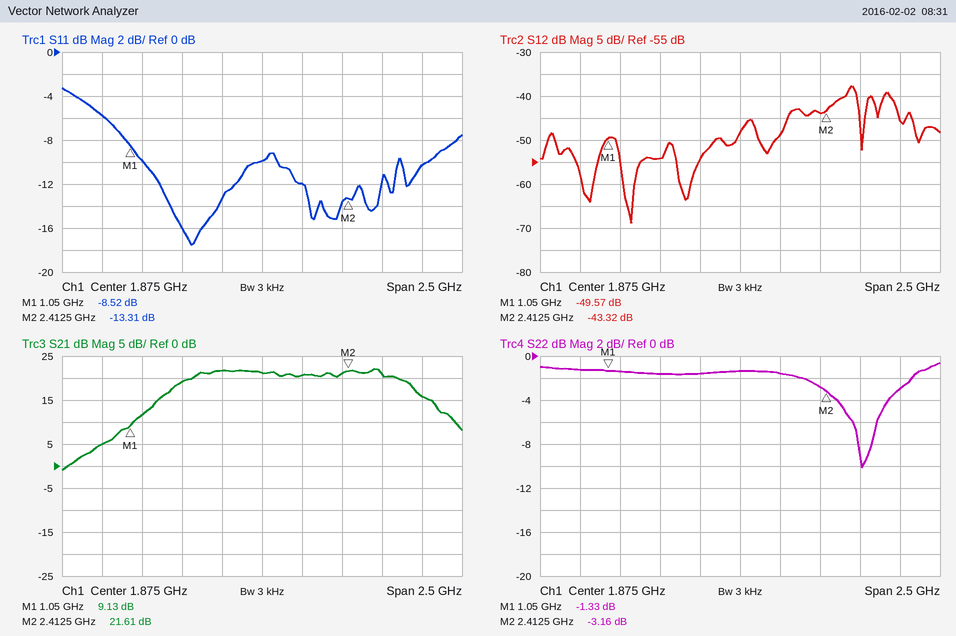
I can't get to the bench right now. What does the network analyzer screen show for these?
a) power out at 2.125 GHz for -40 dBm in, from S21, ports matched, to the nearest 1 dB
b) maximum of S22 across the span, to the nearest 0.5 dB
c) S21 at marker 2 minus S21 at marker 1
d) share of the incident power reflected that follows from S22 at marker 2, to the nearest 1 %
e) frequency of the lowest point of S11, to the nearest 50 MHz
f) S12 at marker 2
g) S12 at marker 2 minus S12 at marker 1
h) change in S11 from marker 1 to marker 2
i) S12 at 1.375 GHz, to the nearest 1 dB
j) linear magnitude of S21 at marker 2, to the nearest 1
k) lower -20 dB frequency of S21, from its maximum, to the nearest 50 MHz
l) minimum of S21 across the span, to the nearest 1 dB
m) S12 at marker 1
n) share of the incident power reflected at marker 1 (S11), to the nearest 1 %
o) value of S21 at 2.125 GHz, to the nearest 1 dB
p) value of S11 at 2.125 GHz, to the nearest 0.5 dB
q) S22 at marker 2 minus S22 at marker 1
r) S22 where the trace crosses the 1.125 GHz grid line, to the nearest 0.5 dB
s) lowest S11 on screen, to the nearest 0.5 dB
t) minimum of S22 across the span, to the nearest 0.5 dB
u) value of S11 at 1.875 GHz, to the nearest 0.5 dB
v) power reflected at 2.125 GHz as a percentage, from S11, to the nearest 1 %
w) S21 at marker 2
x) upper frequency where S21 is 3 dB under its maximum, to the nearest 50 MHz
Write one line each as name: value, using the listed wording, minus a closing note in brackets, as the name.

power out at 2.125 GHz for -40 dBm in, from S21, ports matched, to the nearest 1 dB: -19 dBm
maximum of S22 across the span, to the nearest 0.5 dB: -0.5 dB
S21 at marker 2 minus S21 at marker 1: 12.48 dB
share of the incident power reflected that follows from S22 at marker 2, to the nearest 1 %: 48 %
frequency of the lowest point of S11, to the nearest 50 MHz: 1.45 GHz
S12 at marker 2: -43.32 dB
S12 at marker 2 minus S12 at marker 1: 6.25 dB
change in S11 from marker 1 to marker 2: -4.79 dB
S12 at 1.375 GHz, to the nearest 1 dB: -54 dB
linear magnitude of S21 at marker 2, to the nearest 1: 12
lower -20 dB frequency of S21, from its maximum, to the nearest 50 MHz: 750 MHz
minimum of S21 across the span, to the nearest 1 dB: -1 dB
S12 at marker 1: -49.57 dB
share of the incident power reflected at marker 1 (S11), to the nearest 1 %: 14 %
value of S21 at 2.125 GHz, to the nearest 1 dB: 21 dB
value of S11 at 2.125 GHz, to the nearest 0.5 dB: -12.0 dB
S22 at marker 2 minus S22 at marker 1: -1.83 dB
S22 where the trace crosses the 1.125 GHz grid line, to the nearest 0.5 dB: -1.5 dB
lowest S11 on screen, to the nearest 0.5 dB: -17.5 dB
minimum of S22 across the span, to the nearest 0.5 dB: -10.0 dB
value of S11 at 1.875 GHz, to the nearest 0.5 dB: -10.0 dB
power reflected at 2.125 GHz as a percentage, from S11, to the nearest 1 %: 6 %
S21 at marker 2: 21.61 dB
upper frequency where S21 is 3 dB under its maximum, to the nearest 50 MHz: 2.80 GHz
